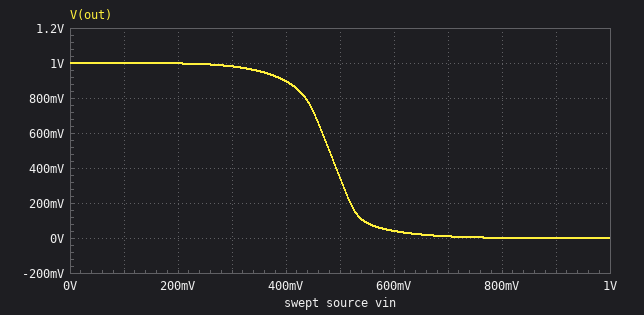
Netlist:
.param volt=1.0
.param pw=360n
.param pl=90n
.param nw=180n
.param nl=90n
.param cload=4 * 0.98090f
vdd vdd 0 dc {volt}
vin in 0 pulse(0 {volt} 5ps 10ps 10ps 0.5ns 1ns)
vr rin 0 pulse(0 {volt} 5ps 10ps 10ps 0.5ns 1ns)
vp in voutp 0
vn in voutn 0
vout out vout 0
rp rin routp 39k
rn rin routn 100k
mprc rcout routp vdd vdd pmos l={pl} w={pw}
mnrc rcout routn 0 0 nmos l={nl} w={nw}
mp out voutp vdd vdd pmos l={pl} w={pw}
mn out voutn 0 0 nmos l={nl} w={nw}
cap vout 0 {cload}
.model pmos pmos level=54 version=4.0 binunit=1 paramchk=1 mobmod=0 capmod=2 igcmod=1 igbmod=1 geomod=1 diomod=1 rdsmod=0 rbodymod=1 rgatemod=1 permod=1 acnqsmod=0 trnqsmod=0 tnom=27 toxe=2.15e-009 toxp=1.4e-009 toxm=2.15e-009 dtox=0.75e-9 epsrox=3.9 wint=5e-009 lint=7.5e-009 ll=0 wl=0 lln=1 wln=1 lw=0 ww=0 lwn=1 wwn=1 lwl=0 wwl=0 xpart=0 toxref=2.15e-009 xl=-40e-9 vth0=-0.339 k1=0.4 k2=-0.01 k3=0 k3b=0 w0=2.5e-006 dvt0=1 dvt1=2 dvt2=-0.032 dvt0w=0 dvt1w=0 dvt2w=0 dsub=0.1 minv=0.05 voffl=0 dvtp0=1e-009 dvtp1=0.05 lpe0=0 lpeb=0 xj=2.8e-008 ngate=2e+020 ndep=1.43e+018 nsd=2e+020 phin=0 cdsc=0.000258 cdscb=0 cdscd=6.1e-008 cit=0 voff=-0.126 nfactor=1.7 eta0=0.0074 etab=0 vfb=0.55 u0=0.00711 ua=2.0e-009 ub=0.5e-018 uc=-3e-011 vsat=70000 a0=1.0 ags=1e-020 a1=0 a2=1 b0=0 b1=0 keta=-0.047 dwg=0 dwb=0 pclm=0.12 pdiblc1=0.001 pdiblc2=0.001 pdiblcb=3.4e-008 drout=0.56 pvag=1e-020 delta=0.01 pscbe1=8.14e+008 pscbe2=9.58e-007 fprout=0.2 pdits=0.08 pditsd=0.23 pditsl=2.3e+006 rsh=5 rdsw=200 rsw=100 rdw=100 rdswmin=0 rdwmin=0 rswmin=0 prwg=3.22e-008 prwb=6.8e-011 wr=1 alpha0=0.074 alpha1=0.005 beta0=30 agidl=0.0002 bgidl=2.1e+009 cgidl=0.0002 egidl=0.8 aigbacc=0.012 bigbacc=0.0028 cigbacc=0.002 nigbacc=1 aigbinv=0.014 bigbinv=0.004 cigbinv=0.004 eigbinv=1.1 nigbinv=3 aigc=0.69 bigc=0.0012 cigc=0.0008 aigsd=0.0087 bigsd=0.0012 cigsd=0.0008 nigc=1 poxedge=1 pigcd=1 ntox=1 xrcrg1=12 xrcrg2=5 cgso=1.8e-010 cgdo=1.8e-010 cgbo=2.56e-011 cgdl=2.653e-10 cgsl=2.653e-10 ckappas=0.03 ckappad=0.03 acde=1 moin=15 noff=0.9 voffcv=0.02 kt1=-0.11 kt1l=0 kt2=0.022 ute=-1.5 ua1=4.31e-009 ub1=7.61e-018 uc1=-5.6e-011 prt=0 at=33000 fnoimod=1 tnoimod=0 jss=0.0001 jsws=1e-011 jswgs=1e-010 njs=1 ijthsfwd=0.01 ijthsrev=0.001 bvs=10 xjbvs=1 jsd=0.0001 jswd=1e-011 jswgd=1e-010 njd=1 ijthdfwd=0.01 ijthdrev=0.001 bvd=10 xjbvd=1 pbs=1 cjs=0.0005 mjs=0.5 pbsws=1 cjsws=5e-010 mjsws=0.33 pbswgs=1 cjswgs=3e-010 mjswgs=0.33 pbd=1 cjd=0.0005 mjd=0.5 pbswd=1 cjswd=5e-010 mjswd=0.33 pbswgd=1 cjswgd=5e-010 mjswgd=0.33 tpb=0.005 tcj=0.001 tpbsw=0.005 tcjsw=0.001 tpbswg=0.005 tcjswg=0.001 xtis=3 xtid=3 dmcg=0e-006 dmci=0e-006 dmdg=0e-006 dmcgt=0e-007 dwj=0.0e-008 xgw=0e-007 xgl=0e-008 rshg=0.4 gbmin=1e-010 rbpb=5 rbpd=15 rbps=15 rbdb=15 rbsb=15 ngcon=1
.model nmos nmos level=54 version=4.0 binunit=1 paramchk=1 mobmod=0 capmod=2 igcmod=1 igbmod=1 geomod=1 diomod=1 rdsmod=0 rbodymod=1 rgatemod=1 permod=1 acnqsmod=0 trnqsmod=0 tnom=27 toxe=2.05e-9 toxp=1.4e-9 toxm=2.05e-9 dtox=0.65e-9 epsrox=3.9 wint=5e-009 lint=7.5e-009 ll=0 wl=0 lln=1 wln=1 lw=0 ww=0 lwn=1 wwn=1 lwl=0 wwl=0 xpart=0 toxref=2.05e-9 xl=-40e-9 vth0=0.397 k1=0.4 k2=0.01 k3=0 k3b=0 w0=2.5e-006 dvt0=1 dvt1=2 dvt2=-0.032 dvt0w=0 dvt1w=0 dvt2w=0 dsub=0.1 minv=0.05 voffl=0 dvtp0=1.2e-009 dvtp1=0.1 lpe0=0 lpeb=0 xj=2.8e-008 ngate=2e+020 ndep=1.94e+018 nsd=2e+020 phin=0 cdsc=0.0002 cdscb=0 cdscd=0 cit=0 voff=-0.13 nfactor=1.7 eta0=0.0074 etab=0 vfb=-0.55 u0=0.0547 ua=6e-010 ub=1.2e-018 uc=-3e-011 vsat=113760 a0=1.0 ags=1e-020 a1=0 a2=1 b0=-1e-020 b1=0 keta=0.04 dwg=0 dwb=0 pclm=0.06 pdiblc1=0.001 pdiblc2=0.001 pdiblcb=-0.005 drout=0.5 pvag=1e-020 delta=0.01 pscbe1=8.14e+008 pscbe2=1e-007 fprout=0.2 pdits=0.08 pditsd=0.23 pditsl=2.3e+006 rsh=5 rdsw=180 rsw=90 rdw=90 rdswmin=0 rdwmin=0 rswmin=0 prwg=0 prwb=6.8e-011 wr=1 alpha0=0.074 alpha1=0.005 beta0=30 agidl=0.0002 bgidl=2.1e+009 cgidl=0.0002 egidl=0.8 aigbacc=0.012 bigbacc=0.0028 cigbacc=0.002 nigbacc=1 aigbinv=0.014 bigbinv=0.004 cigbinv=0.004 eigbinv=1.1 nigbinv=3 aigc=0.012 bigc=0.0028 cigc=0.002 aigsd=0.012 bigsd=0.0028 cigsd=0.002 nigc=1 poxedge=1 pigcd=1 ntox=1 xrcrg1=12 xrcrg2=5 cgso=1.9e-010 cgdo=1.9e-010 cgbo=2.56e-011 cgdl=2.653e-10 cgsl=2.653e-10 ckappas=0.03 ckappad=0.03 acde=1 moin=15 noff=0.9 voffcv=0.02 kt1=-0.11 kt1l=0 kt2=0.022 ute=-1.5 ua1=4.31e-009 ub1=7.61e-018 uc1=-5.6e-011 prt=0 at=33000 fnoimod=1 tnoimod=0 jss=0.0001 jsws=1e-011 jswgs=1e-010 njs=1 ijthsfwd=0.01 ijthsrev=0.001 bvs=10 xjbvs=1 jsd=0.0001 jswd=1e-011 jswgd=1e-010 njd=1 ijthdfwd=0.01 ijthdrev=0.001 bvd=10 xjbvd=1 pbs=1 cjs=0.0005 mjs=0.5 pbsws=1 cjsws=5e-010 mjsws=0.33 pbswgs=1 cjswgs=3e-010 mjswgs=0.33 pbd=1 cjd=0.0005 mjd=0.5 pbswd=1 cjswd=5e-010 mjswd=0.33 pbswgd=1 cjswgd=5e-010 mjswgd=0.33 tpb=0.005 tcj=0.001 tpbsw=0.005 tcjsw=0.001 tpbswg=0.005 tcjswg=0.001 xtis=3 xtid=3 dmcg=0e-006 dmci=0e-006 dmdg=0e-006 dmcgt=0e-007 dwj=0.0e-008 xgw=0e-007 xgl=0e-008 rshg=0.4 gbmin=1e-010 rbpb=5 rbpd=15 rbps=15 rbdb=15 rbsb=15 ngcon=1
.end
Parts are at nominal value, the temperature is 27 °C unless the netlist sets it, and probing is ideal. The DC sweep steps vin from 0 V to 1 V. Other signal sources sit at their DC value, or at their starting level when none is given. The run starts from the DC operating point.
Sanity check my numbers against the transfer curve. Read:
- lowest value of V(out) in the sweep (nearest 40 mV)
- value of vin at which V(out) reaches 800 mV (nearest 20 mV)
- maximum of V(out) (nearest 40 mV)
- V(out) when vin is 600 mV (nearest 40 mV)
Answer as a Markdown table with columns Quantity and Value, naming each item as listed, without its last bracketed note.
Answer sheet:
| Quantity | Value |
|---|---|
| lowest value of V(out) in the sweep | 0 V |
| value of vin at which V(out) reaches 800 mV | 440 mV |
| maximum of V(out) | 1.00 V |
| V(out) when vin is 600 mV | 40 mV |
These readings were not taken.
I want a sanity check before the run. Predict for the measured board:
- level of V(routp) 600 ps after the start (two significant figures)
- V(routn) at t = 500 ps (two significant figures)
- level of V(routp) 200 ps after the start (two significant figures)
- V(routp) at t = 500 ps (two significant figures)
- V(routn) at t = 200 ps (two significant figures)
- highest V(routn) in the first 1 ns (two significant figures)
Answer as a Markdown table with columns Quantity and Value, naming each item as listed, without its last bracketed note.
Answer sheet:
| Quantity | Value |
|---|---|
| level of V(routp) 600 ps after the start | 70 mV |
| V(routn) at t = 500 ps | 1.0 V |
| level of V(routp) 200 ps after the start | 1.0 V |
| V(routp) at t = 500 ps | 1.0 V |
| V(routn) at t = 200 ps | 1.0 V |
| highest V(routn) in the first 1 ns | 1.0 V |
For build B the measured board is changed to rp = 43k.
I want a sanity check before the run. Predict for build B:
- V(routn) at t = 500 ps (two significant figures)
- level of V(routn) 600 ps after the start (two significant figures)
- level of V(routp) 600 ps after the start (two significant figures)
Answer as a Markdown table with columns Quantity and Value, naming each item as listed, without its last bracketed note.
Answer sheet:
| Quantity | Value |
|---|---|
| V(routn) at t = 500 ps | 1.0 V |
| level of V(routn) 600 ps after the start | 49 mV |
| level of V(routp) 600 ps after the start | 89 mV |
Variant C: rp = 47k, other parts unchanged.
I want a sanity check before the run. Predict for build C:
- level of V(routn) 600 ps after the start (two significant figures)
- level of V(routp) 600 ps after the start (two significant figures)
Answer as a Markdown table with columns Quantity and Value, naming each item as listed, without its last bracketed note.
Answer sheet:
| Quantity | Value |
|---|---|
| level of V(routn) 600 ps after the start | 50 mV |
| level of V(routp) 600 ps after the start | 110 mV |
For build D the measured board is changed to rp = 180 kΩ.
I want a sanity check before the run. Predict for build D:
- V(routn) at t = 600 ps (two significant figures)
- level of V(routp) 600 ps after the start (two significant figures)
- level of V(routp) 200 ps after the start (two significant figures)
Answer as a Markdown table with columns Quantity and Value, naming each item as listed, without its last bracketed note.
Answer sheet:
| Quantity | Value |
|---|---|
| V(routn) at t = 600 ps | 120 mV |
| level of V(routp) 600 ps after the start | 550 mV |
| level of V(routp) 200 ps after the start | 810 mV |
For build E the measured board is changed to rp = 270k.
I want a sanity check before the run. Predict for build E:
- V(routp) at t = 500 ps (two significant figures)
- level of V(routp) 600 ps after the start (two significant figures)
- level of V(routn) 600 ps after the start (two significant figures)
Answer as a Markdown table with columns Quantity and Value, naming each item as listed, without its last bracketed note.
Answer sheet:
| Quantity | Value |
|---|---|
| V(routp) at t = 500 ps | 980 mV |
| level of V(routp) 600 ps after the start | 610 mV |
| level of V(routn) 600 ps after the start | 110 mV |
